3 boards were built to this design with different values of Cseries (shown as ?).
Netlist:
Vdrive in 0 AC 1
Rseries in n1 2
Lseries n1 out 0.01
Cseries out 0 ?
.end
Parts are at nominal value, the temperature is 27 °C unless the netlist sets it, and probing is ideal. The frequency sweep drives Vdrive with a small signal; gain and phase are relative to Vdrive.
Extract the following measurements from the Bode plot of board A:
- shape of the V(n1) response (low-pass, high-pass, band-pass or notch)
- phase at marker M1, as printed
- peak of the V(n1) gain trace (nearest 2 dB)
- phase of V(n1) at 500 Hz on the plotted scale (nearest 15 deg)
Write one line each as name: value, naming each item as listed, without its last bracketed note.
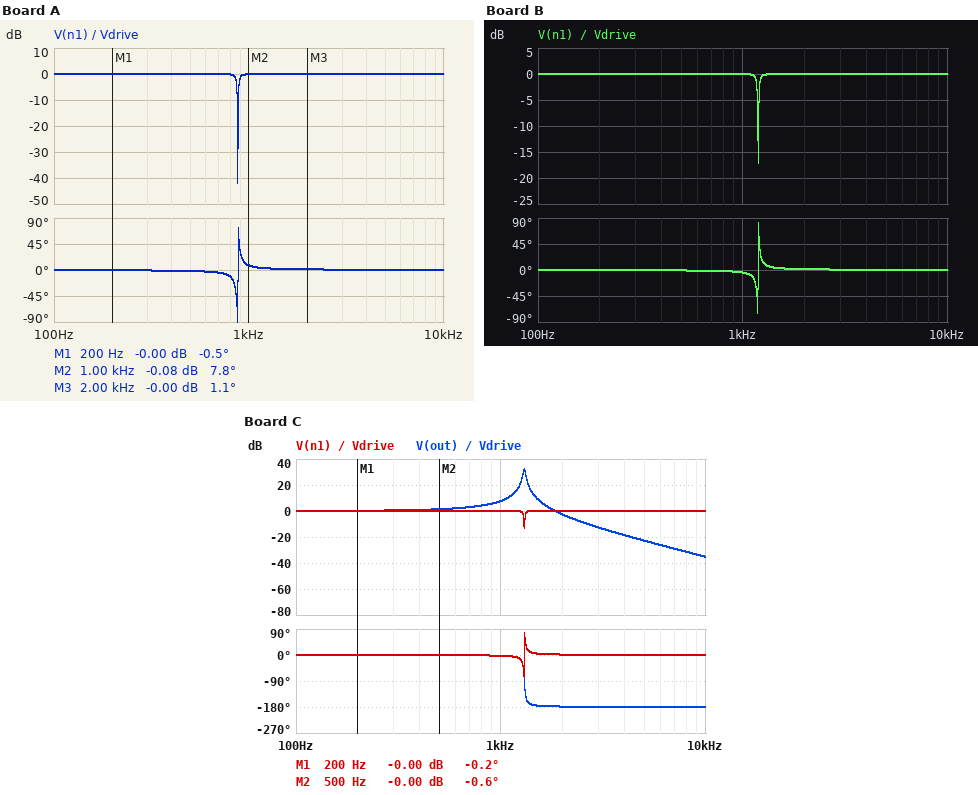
shape of the V(n1) response: notch
phase at marker M1, as printed: -0.5 deg
peak of the V(n1) gain trace: 0 dB
phase of V(n1) at 500 Hz on the plotted scale: 0 deg
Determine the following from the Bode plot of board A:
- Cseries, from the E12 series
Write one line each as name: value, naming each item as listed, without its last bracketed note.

Cseries, from the E12 series: 3.3 µF
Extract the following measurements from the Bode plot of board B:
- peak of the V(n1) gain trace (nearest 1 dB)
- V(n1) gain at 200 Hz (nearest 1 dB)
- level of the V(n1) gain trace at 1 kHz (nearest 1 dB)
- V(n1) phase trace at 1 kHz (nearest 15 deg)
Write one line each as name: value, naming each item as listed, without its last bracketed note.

peak of the V(n1) gain trace: 0 dB
V(n1) gain at 200 Hz: 0 dB
level of the V(n1) gain trace at 1 kHz: 0 dB
V(n1) phase trace at 1 kHz: 0 deg
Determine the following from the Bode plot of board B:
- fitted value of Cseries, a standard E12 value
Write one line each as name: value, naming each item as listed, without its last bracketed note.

fitted value of Cseries, a standard E12 value: 1.8 µF
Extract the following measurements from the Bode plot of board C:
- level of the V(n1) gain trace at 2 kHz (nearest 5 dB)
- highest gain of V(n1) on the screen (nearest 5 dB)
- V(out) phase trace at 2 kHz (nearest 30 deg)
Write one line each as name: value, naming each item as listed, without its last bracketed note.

level of the V(n1) gain trace at 2 kHz: 0 dB
highest gain of V(n1) on the screen: 0 dB
V(out) phase trace at 2 kHz: -180 deg
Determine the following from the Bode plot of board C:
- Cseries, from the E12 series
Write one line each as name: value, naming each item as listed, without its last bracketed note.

Cseries, from the E12 series: 1.5 µF
